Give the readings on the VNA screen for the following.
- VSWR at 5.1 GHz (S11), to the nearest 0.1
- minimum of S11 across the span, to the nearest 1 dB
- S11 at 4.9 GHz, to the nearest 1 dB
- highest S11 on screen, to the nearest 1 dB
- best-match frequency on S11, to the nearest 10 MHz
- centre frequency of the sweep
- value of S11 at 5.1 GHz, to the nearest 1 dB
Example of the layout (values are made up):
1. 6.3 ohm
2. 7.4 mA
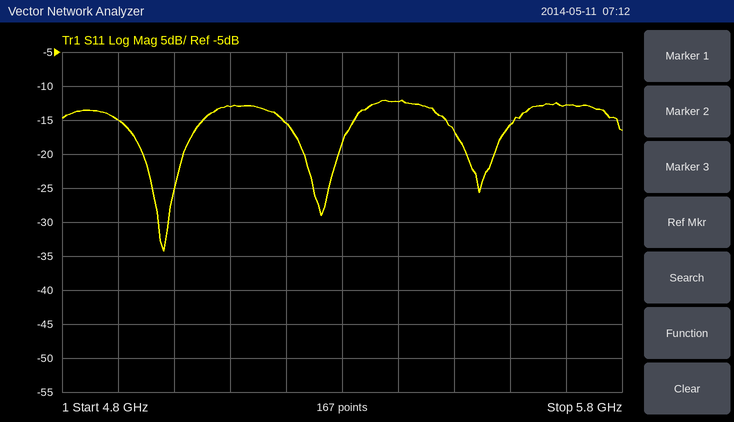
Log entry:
1. 1.6
2. -34 dB
3. -15 dB
4. -12 dB
5. 4.98 GHz
6. 5.3 GHz
7. -13 dB
